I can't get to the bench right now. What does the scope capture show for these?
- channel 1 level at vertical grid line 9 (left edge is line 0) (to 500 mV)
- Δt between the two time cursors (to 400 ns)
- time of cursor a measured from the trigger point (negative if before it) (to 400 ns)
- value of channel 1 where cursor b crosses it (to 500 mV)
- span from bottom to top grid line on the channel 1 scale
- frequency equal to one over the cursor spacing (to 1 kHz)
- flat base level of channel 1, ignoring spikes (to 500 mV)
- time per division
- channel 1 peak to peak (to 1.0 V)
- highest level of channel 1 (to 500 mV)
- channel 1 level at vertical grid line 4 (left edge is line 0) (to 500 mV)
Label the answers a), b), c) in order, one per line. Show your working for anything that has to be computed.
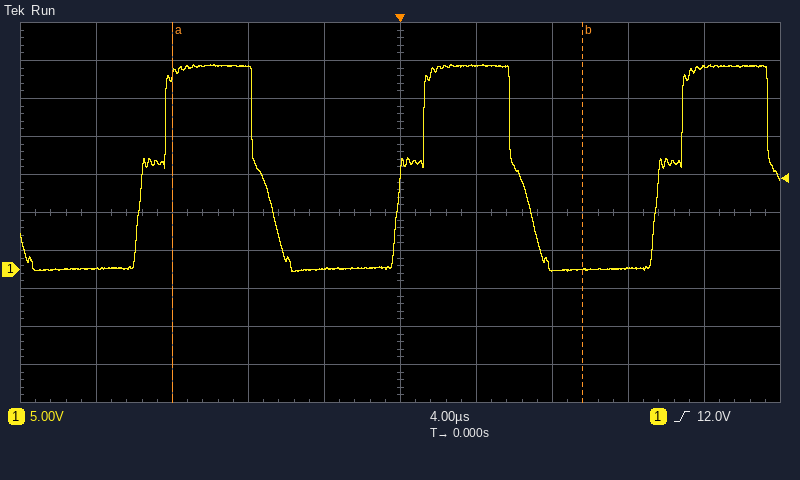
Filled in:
a) 26.5 V
b) 21.6 µs
c) -12.0 µs
d) 0.0 V
e) 50 V
f) 1 / 21.6 µs ≈ 46 kHz
g) 0.0 V
h) 4 µs
i) 27.0 V
j) 27.0 V
k) 0.0 V
